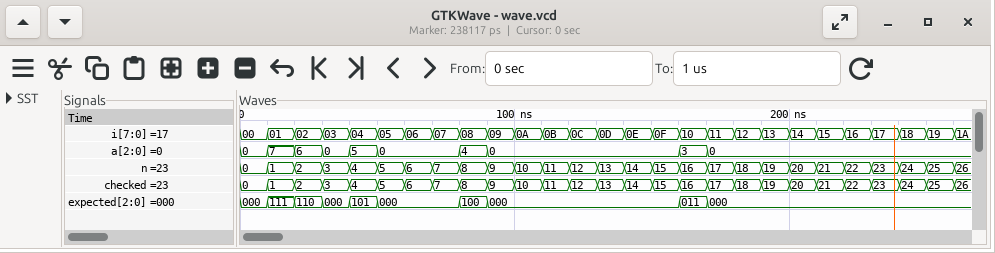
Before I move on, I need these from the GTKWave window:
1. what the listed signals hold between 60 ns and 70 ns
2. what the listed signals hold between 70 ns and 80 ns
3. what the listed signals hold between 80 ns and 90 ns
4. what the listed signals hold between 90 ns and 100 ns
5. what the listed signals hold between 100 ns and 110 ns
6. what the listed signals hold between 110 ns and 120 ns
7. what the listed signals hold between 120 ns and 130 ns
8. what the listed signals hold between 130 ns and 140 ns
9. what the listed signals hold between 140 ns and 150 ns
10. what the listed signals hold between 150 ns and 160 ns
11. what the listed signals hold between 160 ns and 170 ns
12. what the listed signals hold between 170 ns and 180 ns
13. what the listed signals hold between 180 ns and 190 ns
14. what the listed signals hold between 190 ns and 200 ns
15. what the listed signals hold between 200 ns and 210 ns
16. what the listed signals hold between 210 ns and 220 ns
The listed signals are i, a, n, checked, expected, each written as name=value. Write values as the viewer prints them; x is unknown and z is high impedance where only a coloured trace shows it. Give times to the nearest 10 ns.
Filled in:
i=06, a=0, n=6, checked=6, expected=000
i=07, a=0, n=7, checked=7, expected=000
i=08, a=4, n=8, checked=8, expected=100
i=09, a=0, n=9, checked=9, expected=000
i=0A, a=0, n=10, checked=10, expected=000
i=0B, a=0, n=11, checked=11, expected=000
i=0C, a=0, n=12, checked=12, expected=000
i=0D, a=0, n=13, checked=13, expected=000
i=0E, a=0, n=14, checked=14, expected=000
i=0F, a=0, n=15, checked=15, expected=000
i=10, a=3, n=16, checked=16, expected=011
i=11, a=0, n=17, checked=17, expected=000
i=12, a=0, n=18, checked=18, expected=000
i=13, a=0, n=19, checked=19, expected=000
i=14, a=0, n=20, checked=20, expected=000
i=15, a=0, n=21, checked=21, expected=000
